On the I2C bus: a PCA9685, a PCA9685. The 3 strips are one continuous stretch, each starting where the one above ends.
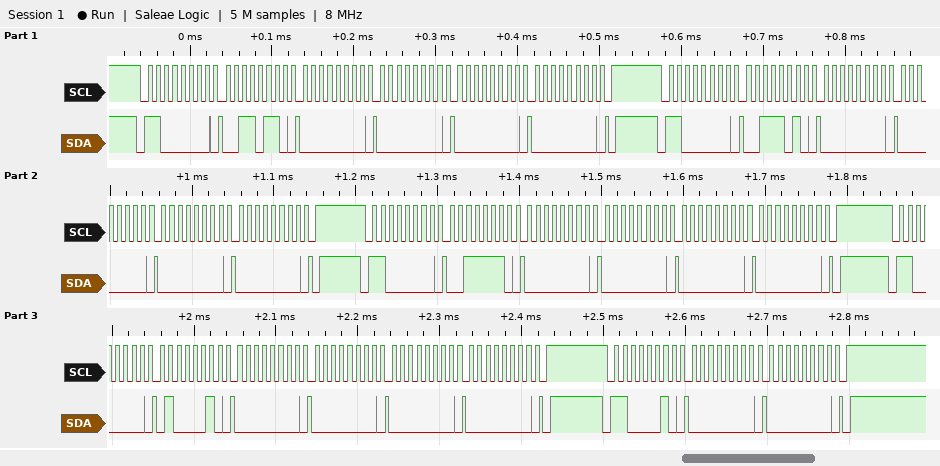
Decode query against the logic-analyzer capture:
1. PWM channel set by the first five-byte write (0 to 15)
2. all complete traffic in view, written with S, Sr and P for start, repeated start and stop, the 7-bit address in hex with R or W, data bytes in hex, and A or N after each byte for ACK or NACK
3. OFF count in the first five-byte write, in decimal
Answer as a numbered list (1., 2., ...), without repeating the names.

1. 12
2. S 60W A 36 A 00 A 00 A 00 A 00 A P S 60W A 3A A 00 A 00 A 00 A 00 A P S 60W A 3E A 00 A 00 A 00 A 00 A P S 60W A 42 A 00 A 00 A 00 A 00 A P S 61W A 00 A 00 A P
3. 0
